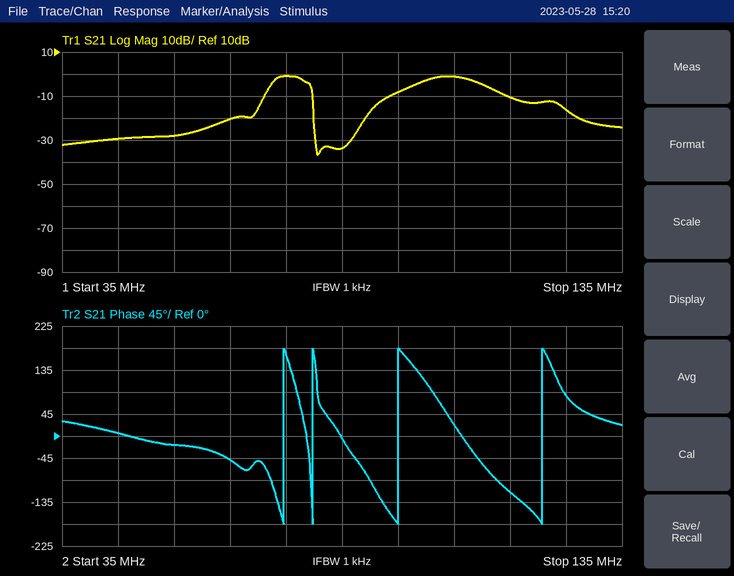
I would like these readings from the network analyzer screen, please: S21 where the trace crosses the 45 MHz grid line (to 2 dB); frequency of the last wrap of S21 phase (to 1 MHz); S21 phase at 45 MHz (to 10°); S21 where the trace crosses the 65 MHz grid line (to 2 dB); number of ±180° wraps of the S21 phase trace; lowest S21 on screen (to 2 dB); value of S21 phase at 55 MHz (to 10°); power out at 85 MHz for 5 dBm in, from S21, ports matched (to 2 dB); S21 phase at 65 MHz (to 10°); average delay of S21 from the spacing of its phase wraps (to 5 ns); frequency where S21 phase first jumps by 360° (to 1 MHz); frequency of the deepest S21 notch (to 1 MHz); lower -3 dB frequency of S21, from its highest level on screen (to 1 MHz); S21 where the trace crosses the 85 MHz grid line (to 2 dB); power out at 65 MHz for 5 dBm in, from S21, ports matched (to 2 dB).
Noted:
-30 dB
121 MHz
10°
-20 dB
4
-36 dB
-20°
-28 dBm
-50°
65 ns
75 MHz
81 MHz
73 MHz
-34 dB
-16 dBm
